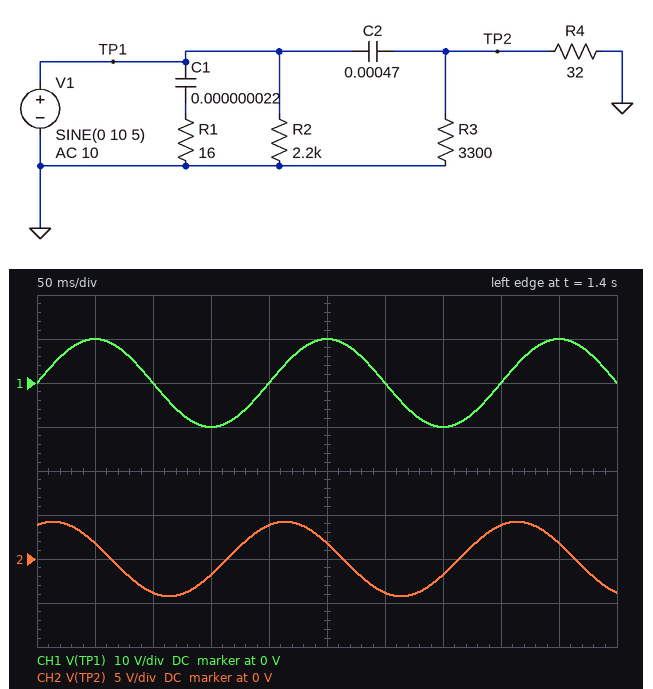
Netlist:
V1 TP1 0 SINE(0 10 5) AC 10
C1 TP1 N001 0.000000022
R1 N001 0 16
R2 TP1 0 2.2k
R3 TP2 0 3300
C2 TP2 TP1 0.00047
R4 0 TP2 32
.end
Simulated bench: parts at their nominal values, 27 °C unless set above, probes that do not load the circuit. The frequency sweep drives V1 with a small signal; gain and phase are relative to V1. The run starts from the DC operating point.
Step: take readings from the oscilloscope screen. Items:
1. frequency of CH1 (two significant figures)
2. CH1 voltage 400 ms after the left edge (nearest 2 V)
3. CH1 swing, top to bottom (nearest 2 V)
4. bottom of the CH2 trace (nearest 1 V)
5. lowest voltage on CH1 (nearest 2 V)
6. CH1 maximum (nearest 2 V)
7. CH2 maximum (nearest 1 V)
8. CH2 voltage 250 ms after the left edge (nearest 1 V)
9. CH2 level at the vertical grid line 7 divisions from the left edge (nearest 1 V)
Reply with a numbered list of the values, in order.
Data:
1. 5.0 Hz
2. 0 V
3. 20 V
4. -4 V
5. -10 V
6. 10 V
7. 4 V
8. 2 V
9. -2 V
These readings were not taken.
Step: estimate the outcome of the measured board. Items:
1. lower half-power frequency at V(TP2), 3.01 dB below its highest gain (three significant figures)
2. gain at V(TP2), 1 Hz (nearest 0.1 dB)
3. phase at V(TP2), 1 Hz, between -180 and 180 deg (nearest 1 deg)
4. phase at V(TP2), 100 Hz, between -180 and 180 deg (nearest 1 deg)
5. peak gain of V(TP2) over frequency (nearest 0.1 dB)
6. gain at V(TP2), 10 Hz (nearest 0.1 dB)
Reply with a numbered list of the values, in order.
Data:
1. 10.7 Hz
2. -20.6 dB
3. 85 deg
4. 6 deg
5. 0 dB
6. -3.3 dB
